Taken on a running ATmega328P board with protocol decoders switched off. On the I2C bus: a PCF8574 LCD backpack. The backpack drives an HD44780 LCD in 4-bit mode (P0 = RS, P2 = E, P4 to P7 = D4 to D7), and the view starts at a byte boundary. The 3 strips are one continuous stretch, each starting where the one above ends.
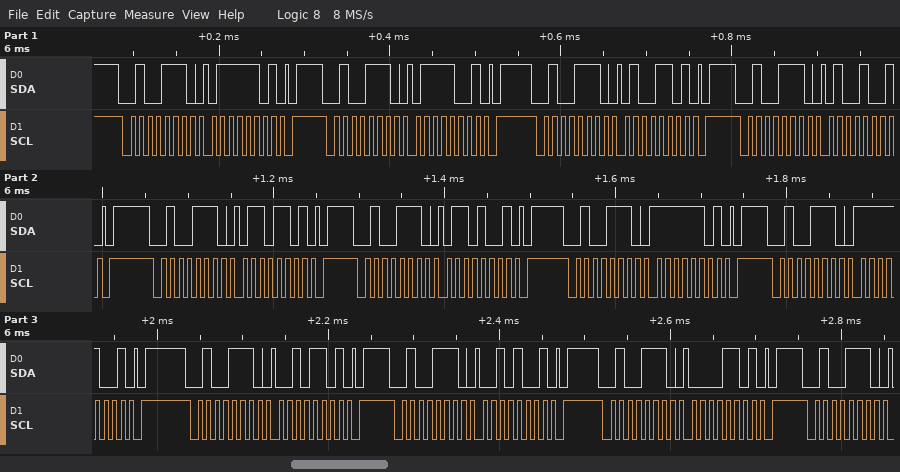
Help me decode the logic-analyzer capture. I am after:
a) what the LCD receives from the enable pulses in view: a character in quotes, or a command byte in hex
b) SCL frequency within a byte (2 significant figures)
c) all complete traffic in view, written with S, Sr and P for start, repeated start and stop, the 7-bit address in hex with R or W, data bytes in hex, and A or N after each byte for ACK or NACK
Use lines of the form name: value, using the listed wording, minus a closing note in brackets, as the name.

what the LCD receives from the enable pulses in view: a character in quotes, or a command byte in hex: 't' 'o'
SCL frequency within a byte: 100 kHz
all complete traffic in view, written with S, Sr and P for start, repeated start and stop, the 7-bit address in hex with R or W, data bytes in hex, and A or N after each byte for ACK or NACK: S 27W A 7D A P S 27W A 79 A P S 27W A 4D A P S 27W A 49 A P S 27W A 6D A P S 27W A 69 A P S 27W A FD A P S 27W A F9 A P S 27W A 2D A P S 27W A 29 A P S 27W A 0D A P S 27W A
